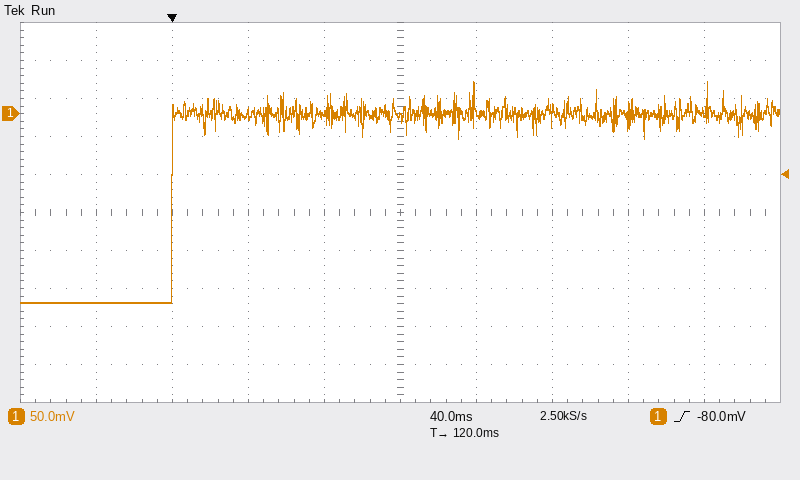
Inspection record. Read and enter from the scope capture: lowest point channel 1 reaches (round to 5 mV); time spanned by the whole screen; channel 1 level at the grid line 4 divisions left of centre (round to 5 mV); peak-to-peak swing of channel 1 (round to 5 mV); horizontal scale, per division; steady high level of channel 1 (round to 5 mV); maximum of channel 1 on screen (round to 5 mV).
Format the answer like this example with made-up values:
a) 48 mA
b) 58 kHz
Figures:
a) -250 mV
b) 400 ms
c) -250 mV
d) 290 mV
e) 40 ms
f) 0 mV
g) 40 mV
